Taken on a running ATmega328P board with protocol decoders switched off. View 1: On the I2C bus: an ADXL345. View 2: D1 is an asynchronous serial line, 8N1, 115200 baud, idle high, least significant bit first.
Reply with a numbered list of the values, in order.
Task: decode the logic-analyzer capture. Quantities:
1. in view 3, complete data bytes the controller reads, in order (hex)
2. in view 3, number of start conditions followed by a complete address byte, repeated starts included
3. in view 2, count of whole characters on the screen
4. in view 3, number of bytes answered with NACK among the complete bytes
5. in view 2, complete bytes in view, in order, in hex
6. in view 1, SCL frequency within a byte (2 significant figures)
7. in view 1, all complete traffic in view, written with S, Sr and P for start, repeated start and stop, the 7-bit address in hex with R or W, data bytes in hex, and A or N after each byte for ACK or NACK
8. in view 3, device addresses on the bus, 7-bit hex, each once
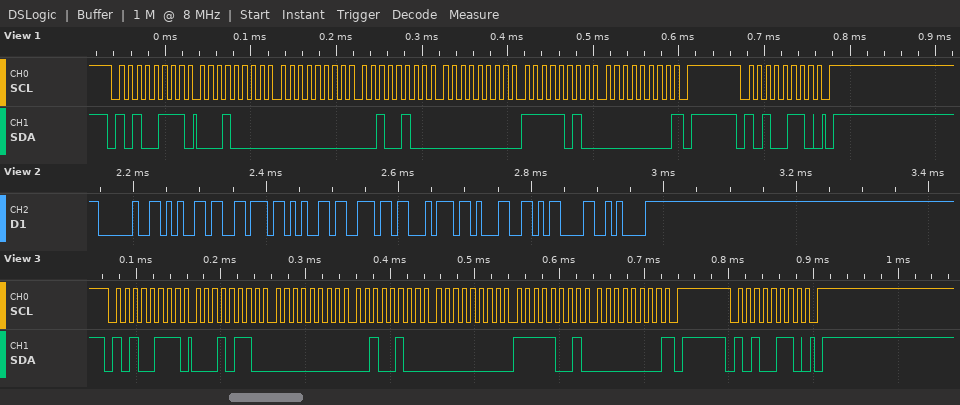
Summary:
1. 16 00 24 00 F9 00
2. 2
3. 9
4. 1
5. 20 65 76 65 6E 74 31 0D 0A
6. 100 kHz
7. S 53R A 10 A 00 A 24 A 00 A FA A 00 N P S 53W A P
8. 0x53
